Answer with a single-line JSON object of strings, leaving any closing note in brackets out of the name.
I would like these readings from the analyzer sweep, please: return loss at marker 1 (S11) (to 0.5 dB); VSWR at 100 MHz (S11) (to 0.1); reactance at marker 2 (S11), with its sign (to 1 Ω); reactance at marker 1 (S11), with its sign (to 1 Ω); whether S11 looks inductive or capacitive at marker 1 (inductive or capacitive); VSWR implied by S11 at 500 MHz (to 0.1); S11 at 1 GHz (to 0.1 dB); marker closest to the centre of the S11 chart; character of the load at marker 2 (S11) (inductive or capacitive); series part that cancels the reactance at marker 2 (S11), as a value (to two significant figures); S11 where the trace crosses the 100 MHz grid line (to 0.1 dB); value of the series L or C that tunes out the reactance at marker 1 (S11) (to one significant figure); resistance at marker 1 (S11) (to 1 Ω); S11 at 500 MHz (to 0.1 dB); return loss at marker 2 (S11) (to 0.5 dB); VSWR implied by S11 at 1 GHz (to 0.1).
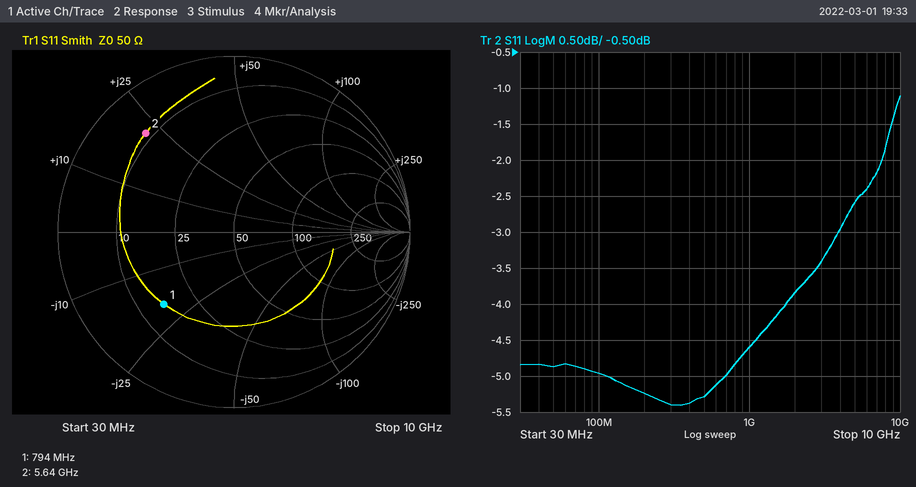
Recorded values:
{"return loss at marker 1 (S11)": "5.0 dB", "VSWR at 100 MHz (S11)": "3.6", "reactance at marker 2 (S11), with its sign": "+22 Ω", "reactance at marker 1 (S11), with its sign": "-19 Ω", "whether S11 looks inductive or capacitive at marker 1": "capacitive", "VSWR implied by S11 at 500 MHz": "3.4", "S11 at 1 GHz": "-4.6 dB", "marker closest to the centre of the S11 chart": "marker 1", "character of the load at marker 2 (S11)": "inductive", "series part that cancels the reactance at marker 2 (S11), as a value": "1.3 pF", "S11 where the trace crosses the 100 MHz grid line": "-5.0 dB", "value of the series L or C that tunes out the reactance at marker 1 (S11)": "4 nH", "resistance at marker 1 (S11)": "16 Ω", "S11 at 500 MHz": "-5.3 dB", "return loss at marker 2 (S11)": "2.5 dB", "VSWR implied by S11 at 1 GHz": "3.9"}
